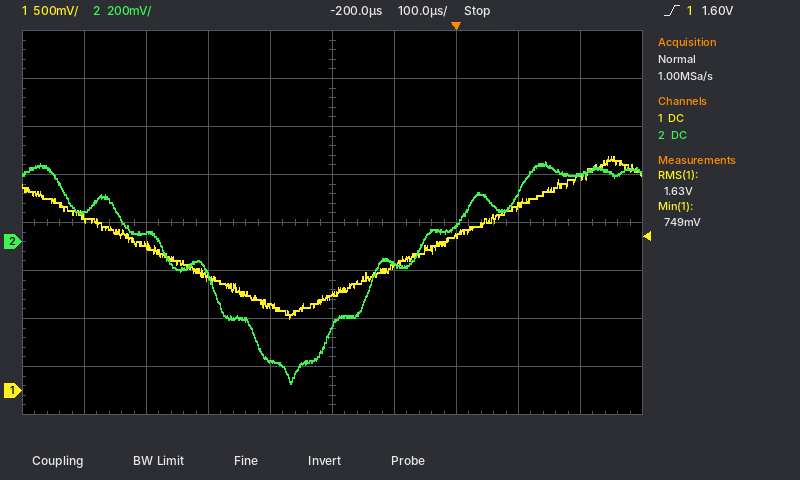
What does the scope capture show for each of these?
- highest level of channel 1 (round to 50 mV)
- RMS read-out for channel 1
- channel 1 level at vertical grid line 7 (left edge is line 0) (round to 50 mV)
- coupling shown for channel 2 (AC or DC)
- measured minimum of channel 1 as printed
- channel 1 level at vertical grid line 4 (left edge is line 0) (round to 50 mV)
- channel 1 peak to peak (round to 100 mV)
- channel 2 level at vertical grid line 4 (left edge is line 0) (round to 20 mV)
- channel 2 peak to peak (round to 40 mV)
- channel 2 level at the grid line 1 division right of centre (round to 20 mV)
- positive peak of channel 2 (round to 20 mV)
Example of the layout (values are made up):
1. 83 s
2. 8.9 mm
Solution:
1. 2.45 V
2. 1.63 V
3. 1.60 V
4. DC
5. 749 mV
6. 900 mV
7. 1.70 V
8. -500 mV
9. 920 mV
10. -100 mV
11. 340 mV
